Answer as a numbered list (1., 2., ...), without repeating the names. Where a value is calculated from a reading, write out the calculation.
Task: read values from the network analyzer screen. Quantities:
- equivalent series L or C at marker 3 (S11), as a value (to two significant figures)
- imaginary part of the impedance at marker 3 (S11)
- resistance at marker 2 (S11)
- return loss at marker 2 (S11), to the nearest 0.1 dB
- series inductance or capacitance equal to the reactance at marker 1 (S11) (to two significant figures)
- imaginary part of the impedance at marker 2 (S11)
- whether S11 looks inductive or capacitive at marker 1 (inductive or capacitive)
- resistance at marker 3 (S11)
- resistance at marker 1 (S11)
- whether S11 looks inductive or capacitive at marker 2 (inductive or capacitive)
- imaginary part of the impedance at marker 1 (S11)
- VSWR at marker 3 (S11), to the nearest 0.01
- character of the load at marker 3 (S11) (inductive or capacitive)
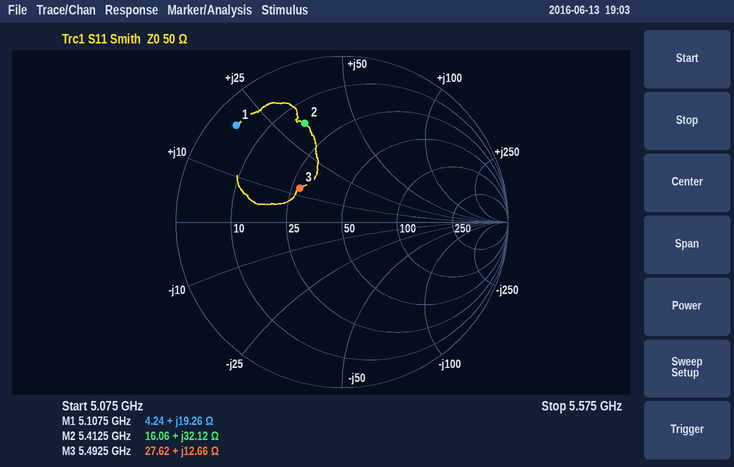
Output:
1. L = 12.66 Ω/(2π × 5.4925 GHz) ≈ 367 pH, so 370 pH to two significant figures
2. +12.66 Ω
3. 16.06 Ω
4. 3.9 dB
5. L = 19.26 Ω/(2π × 5.1075 GHz) ≈ 600 pH
6. +32.12 Ω
7. inductive
8. 27.62 Ω
9. 4.24 Ω
10. inductive
11. +19.26 Ω
12. 1.97
13. inductive
